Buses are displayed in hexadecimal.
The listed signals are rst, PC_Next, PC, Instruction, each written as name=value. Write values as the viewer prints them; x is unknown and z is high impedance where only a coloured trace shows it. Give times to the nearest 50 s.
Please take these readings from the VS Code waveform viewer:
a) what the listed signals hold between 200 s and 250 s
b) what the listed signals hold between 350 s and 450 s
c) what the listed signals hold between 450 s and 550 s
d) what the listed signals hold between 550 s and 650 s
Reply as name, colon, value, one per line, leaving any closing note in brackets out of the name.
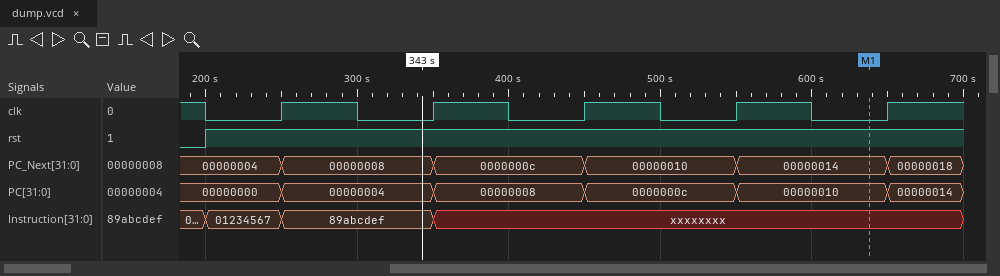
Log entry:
what the listed signals hold between 200 s and 250 s: rst=1, PC_Next=00000004, PC=00000000, Instruction=01234567
what the listed signals hold between 350 s and 450 s: rst=1, PC_Next=0000000c, PC=00000008, Instruction=xxxxxxxx
what the listed signals hold between 450 s and 550 s: rst=1, PC_Next=00000010, PC=0000000c, Instruction=xxxxxxxx
what the listed signals hold between 550 s and 650 s: rst=1, PC_Next=00000014, PC=00000010, Instruction=xxxxxxxx
